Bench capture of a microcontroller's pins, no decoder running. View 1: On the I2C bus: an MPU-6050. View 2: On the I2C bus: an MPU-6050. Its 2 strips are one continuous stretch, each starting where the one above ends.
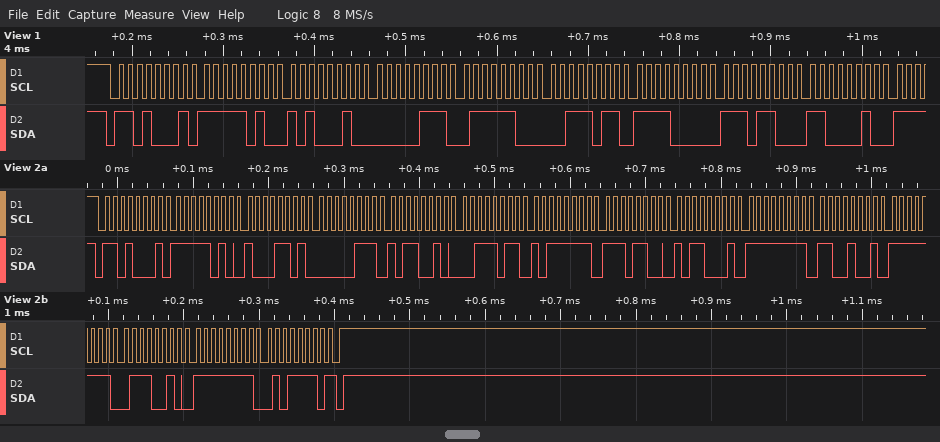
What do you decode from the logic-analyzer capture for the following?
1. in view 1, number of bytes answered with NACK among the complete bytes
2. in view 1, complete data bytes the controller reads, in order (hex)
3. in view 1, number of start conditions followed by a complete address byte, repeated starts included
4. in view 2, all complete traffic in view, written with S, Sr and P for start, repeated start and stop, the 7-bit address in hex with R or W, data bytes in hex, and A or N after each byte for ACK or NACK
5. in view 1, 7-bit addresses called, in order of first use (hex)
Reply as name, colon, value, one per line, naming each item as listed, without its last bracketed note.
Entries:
in view 1, number of bytes answered with NACK among the complete bytes: 0
in view 1, complete data bytes the controller reads, in order: FA A2 07 7C 3B F0 EC C2
in view 1, number of start conditions followed by a complete address byte, repeated starts included: 1
in view 2, all complete traffic in view, written with S, Sr and P for start, repeated start and stop, the 7-bit address in hex with R or W, data bytes in hex, and A or N after each byte for ACK or NACK: S 68R A FA A 8D A 07 A B2 A 3B A BF A EC A B1 A FF A C9 A FF A 72 A FF A 5E N P
in view 1, 7-bit addresses called, in order of first use: 0x68
